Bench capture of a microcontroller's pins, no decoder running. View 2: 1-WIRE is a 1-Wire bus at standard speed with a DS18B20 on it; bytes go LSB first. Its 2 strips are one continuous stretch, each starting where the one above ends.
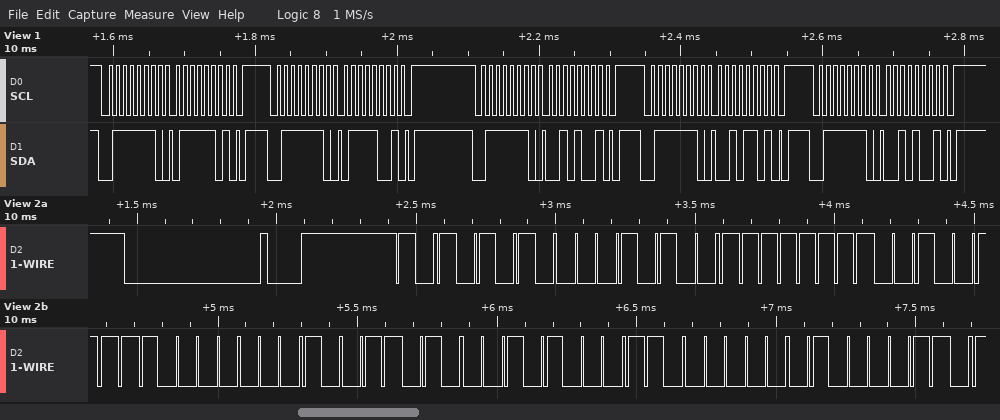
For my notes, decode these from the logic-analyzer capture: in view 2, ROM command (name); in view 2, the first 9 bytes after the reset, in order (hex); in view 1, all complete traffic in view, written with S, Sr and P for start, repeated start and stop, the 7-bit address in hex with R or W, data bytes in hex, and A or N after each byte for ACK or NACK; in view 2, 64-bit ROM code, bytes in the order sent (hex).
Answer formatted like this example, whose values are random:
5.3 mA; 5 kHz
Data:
Match ROM; 55 28 FF E4 01 59 14 03 C2; S 3FW A 7D A P S 3FW A 79 A P S 3FW A 29 A P S 3FW A 2D A P S 3FW A 29 A P; 28 FF E4 01 59 14 03 C2
